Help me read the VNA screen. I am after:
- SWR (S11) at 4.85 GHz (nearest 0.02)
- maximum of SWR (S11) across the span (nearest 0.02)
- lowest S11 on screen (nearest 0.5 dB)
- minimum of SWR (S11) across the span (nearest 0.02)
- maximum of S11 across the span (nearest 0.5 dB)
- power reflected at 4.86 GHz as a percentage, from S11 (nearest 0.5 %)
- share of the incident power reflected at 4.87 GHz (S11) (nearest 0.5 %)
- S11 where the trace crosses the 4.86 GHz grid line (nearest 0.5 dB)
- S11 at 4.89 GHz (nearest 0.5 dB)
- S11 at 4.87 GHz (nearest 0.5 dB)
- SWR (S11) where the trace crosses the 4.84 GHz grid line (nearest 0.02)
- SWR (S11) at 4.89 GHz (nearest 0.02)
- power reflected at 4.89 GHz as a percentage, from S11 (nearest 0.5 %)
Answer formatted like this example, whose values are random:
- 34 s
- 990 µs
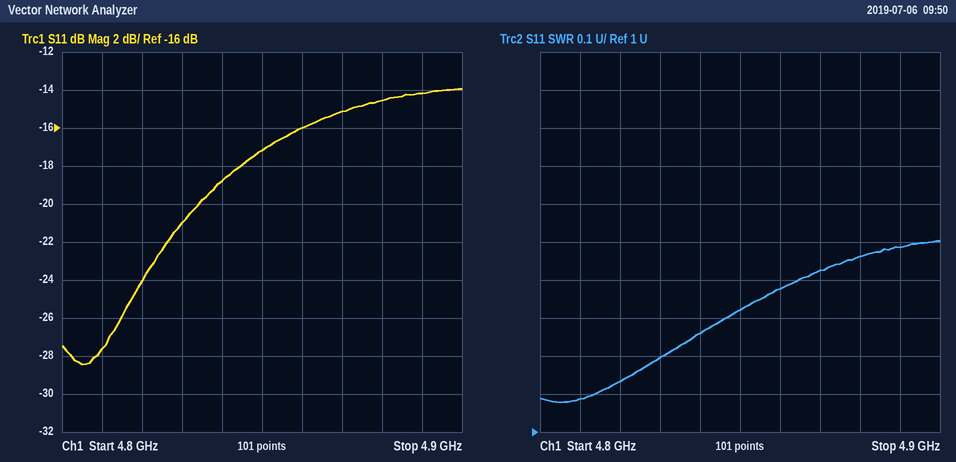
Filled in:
- 1.32
- 1.50
- -28.5 dB
- 1.08
- -14.0 dB
- 2.5 %
- 3.0 %
- -16.0 dB
- -14.0 dB
- -15.0 dB
- 1.26
- 1.48
- 4.0 %
